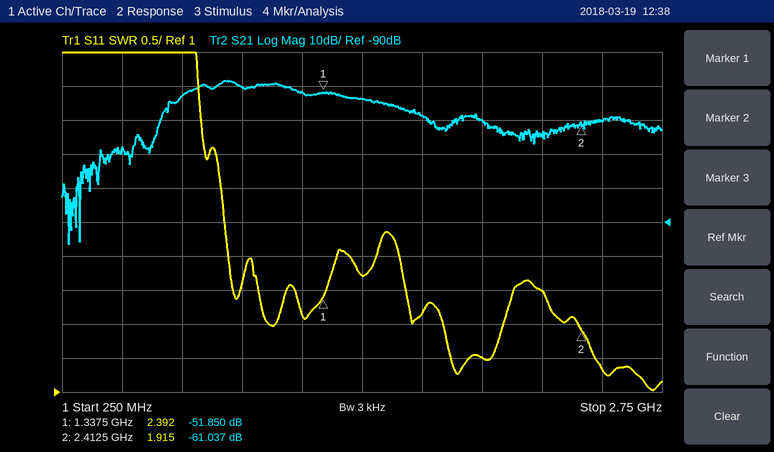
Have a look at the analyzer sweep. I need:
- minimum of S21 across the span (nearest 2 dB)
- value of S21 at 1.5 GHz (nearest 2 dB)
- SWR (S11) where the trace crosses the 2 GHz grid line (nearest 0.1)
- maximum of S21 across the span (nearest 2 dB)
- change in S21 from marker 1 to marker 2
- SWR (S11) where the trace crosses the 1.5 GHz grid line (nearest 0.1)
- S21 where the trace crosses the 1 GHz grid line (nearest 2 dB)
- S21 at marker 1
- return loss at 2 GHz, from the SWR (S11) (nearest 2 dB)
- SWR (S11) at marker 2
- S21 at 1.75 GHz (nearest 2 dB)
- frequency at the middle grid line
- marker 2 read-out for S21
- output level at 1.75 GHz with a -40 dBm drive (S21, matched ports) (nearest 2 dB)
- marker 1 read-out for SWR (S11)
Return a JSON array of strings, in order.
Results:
["-96 dB", "-54 dB", "1.5", "-48 dB", "-9.187 dB", "2.7", "-50 dB", "-51.850 dB", "14 dB", "1.915", "-58 dB", "1.5 GHz", "-61.037 dB", "-98 dBm", "2.392"]
